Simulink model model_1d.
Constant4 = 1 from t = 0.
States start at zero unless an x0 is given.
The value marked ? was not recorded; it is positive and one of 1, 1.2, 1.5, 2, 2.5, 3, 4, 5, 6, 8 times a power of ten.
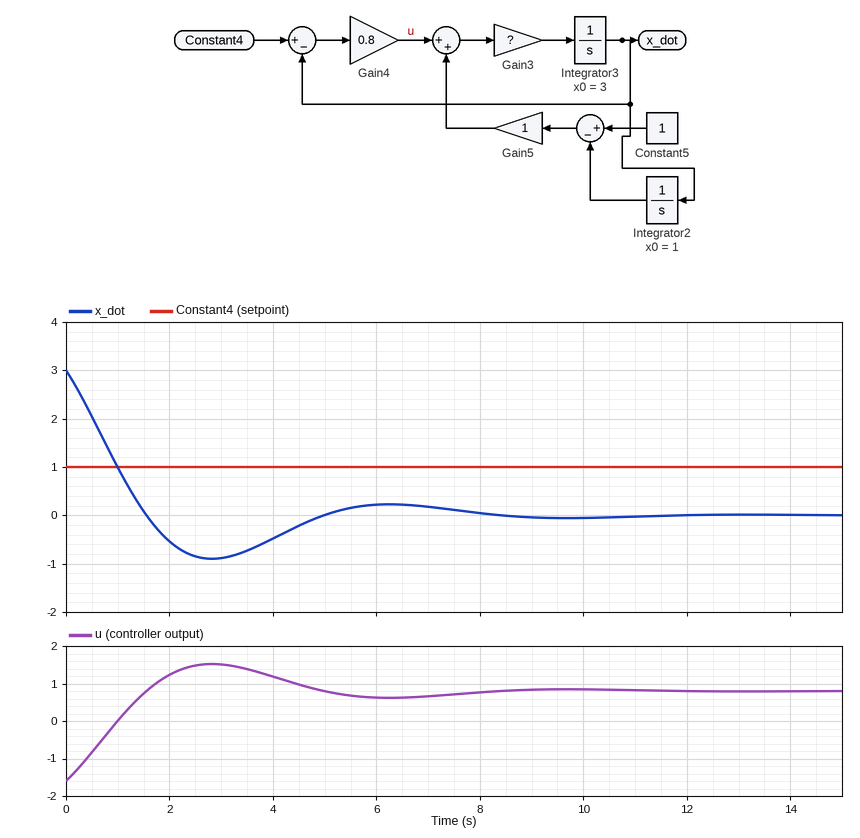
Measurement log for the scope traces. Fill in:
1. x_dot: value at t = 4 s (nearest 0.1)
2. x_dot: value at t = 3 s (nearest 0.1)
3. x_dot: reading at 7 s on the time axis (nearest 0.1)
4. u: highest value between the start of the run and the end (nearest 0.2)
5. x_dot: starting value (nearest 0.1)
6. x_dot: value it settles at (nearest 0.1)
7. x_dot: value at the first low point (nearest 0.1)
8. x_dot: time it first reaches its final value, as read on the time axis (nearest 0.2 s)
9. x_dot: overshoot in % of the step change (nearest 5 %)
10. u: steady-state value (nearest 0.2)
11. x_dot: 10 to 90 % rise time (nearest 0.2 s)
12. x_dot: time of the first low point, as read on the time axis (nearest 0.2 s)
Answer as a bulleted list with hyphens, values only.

- -0.5
- -0.9
- 0.2
- 1.6
- 3.0
- 0.0
- -0.9
- 1.6 s
- 30 %
- 0.8
- 1.2 s
- 2.8 s
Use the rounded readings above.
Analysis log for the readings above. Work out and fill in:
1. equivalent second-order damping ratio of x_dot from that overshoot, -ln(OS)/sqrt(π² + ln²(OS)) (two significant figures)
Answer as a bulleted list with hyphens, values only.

- 0.36
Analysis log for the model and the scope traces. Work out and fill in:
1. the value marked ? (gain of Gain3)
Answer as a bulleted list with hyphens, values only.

- 1
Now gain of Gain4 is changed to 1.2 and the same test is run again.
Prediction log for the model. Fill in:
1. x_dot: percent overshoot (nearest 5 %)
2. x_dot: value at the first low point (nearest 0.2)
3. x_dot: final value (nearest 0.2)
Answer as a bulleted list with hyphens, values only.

- 15 %
- -0.4
- 0.0
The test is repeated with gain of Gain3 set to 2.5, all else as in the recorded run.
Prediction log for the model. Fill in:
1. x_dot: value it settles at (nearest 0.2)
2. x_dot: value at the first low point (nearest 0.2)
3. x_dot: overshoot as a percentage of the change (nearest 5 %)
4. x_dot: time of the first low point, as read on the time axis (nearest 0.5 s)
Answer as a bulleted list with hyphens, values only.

- 0.0
- -0.4
- 15 %
- 2.0 s
